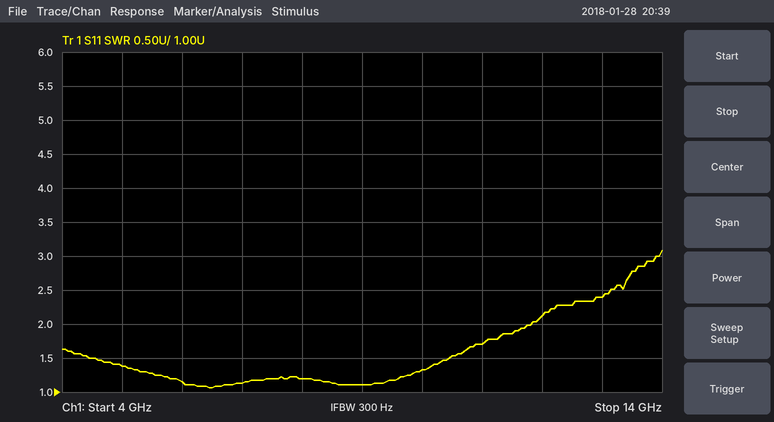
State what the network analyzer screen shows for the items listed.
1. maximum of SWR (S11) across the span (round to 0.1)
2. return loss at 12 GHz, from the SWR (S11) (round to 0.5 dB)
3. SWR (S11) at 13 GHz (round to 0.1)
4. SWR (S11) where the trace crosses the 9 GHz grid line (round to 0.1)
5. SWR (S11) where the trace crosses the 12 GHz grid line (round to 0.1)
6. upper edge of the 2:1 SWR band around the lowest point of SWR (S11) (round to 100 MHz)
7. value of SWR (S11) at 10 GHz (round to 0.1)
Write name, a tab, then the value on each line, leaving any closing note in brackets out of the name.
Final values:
maximum of SWR (S11) across the span	3.1
return loss at 12 GHz, from the SWR (S11)	9.0 dB
SWR (S11) at 13 GHz	2.4
SWR (S11) where the trace crosses the 9 GHz grid line	1.1
SWR (S11) where the trace crosses the 12 GHz grid line	2.1
upper edge of the 2:1 SWR band around the lowest point of SWR (S11)	11.8 GHz
value of SWR (S11) at 10 GHz	1.3
